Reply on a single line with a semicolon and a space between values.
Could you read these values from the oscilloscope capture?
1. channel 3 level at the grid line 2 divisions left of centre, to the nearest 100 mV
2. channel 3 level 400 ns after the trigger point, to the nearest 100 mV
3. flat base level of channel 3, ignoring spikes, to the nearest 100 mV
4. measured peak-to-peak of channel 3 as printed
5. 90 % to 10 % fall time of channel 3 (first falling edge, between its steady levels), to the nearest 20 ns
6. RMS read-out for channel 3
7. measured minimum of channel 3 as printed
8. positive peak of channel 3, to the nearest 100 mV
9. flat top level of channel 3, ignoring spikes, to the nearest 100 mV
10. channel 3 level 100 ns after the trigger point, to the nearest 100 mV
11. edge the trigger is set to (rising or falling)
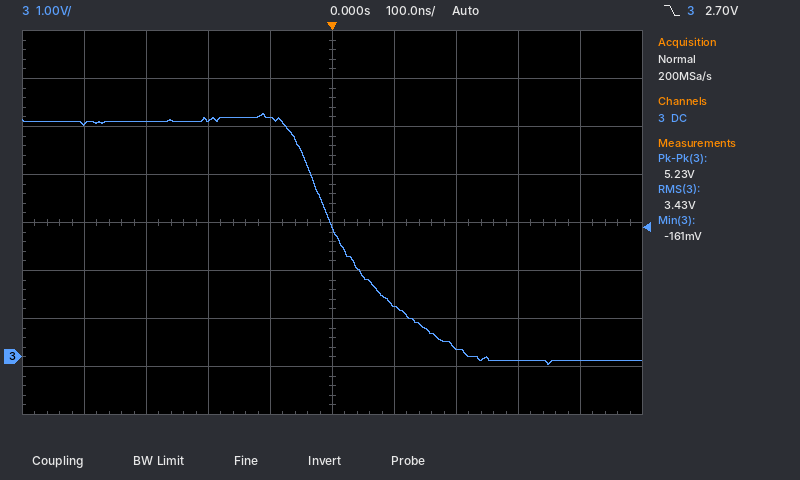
4.9 V; -100 mV; -100 mV; 5.23 V; 220 ns; 3.43 V; -161 mV; 5.1 V; 4.9 V; 1.1 V; falling
